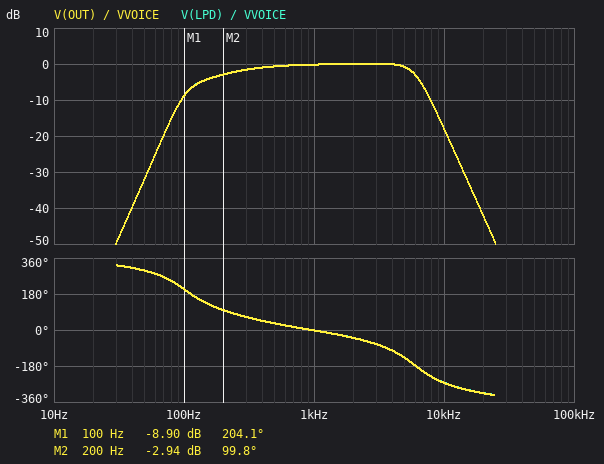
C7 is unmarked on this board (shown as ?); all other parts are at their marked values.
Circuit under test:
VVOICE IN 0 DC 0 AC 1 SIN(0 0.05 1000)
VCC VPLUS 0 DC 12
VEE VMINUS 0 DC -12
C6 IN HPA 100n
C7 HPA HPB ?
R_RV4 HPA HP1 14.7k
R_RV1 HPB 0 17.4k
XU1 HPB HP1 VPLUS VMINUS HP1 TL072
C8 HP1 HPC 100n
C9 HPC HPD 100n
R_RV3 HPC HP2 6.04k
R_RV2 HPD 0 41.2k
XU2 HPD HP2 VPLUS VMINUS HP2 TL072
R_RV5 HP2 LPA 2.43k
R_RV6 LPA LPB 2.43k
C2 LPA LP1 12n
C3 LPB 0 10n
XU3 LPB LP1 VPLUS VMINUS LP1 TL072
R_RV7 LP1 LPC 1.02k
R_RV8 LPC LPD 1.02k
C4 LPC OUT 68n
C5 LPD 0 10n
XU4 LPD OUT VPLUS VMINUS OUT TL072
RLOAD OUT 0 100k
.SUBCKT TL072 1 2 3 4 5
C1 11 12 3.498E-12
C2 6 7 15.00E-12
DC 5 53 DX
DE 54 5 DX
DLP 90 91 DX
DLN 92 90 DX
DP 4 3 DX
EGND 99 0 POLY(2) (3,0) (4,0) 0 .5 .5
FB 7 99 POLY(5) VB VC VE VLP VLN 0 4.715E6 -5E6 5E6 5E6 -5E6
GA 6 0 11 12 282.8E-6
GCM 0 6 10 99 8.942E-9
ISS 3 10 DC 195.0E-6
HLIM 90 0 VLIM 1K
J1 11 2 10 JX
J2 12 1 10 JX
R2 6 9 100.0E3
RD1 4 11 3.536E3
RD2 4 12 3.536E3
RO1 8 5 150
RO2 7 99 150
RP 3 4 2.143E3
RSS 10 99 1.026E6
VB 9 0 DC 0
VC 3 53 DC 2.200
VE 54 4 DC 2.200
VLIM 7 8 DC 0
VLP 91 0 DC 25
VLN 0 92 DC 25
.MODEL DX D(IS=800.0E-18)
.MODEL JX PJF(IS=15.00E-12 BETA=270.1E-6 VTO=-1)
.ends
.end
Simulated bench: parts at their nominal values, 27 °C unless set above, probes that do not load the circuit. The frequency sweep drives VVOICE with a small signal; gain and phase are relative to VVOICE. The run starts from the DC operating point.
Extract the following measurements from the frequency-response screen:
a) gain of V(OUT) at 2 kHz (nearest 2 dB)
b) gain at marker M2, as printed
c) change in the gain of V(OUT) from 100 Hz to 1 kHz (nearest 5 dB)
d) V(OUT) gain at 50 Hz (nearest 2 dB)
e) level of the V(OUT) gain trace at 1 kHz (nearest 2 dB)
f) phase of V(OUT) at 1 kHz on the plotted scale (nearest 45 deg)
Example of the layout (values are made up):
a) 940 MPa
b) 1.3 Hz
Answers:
a) 0 dB
b) -2.94 dB
c) 10 dB
d) -32 dB
e) 0 dB
f) 0 deg
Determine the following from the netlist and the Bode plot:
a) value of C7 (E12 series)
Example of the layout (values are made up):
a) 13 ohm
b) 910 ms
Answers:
a) 39 nF
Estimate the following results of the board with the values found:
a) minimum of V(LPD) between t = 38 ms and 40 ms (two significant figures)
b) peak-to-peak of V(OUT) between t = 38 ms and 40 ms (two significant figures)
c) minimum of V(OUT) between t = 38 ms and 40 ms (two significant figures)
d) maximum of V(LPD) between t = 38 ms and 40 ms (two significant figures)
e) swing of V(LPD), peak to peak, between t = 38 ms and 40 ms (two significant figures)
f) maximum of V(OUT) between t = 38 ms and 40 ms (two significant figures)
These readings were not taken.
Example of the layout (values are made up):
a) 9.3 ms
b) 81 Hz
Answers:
a) -49 mV
b) 98 mV
c) -49 mV
d) 49 mV
e) 98 mV
f) 49 mV
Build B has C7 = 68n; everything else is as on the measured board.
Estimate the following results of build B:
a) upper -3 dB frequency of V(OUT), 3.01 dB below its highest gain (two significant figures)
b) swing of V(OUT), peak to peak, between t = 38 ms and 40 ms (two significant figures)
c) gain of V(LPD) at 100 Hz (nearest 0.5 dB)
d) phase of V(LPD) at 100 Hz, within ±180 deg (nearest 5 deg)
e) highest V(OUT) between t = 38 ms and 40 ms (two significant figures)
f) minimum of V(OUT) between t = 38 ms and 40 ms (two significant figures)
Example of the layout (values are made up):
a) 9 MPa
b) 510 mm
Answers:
a) 6.0 kHz
b) 100 mV
c) -5.0 dB
d) -170 deg
e) 50 mV
f) -50 mV
